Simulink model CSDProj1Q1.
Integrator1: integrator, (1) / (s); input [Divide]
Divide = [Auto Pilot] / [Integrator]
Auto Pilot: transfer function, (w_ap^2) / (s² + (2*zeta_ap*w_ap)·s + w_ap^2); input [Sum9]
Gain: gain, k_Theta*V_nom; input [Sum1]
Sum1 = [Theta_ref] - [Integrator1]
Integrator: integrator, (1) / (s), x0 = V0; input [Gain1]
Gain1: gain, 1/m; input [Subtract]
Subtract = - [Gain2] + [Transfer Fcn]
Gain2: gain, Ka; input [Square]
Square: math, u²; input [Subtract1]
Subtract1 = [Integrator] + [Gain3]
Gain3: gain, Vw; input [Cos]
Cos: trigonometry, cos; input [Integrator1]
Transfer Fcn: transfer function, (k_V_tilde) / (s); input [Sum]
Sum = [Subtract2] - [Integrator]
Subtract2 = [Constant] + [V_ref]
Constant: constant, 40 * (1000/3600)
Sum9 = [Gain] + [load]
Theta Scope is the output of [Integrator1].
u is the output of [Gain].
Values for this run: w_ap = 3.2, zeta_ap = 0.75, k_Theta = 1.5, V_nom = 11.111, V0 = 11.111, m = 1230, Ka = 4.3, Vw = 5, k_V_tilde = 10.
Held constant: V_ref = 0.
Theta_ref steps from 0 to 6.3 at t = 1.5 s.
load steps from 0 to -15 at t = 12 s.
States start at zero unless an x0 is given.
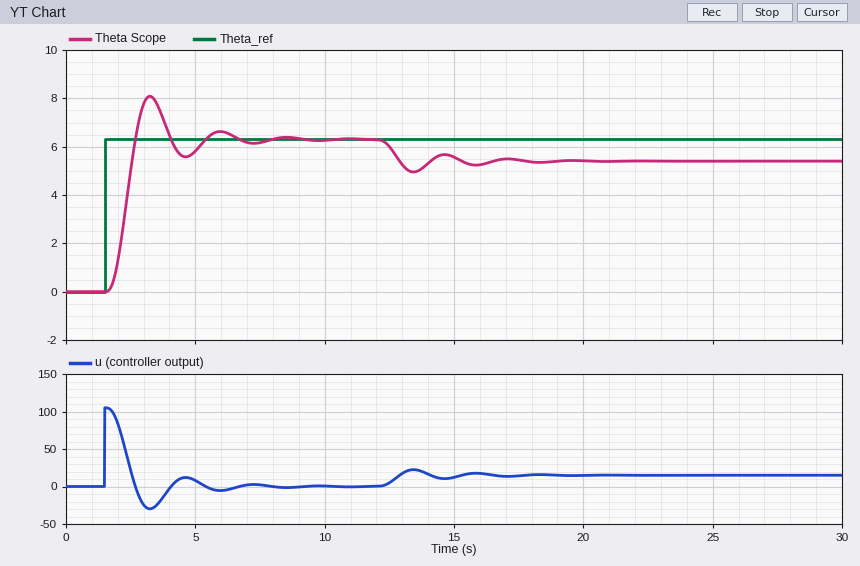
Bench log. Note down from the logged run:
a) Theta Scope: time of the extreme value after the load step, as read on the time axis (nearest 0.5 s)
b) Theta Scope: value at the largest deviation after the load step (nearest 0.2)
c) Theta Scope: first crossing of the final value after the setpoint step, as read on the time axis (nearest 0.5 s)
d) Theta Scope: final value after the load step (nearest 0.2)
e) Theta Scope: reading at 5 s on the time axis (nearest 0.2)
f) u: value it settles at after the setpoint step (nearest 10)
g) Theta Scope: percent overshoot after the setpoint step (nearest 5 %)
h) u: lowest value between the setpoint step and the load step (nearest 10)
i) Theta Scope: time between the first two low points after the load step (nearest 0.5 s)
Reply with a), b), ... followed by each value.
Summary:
a) 13.5 s
b) 5.0
c) 2.5 s
d) 5.4
e) 5.8
f) 0
g) 30 %
h) -30
i) 2.5 s
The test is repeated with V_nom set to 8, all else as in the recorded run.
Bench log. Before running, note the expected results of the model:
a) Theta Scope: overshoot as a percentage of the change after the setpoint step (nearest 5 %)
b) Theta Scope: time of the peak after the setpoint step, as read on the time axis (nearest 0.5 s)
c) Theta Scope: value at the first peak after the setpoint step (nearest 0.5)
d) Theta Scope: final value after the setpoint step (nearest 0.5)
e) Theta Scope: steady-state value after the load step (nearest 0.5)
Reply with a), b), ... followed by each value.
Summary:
a) 15 %
b) 3.5 s
c) 7.0
d) 6.5
e) 5.0
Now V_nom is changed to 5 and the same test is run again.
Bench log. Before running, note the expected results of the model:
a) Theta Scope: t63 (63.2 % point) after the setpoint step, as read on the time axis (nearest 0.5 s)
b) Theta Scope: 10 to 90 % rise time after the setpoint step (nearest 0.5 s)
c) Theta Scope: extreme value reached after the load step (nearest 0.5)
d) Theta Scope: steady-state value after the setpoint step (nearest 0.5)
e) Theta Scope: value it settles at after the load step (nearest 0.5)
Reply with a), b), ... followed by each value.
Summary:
a) 3.0 s
b) 1.5 s
c) 4.0
d) 6.5
e) 4.5
